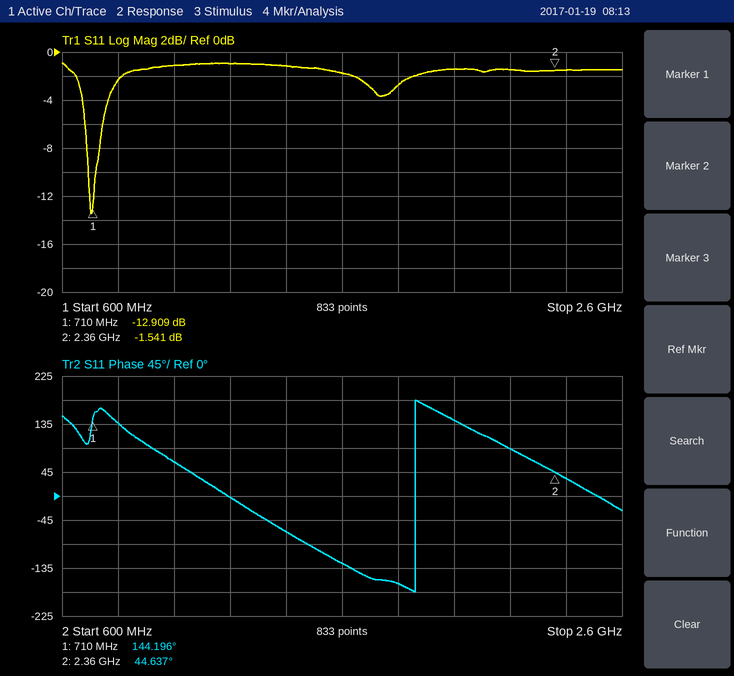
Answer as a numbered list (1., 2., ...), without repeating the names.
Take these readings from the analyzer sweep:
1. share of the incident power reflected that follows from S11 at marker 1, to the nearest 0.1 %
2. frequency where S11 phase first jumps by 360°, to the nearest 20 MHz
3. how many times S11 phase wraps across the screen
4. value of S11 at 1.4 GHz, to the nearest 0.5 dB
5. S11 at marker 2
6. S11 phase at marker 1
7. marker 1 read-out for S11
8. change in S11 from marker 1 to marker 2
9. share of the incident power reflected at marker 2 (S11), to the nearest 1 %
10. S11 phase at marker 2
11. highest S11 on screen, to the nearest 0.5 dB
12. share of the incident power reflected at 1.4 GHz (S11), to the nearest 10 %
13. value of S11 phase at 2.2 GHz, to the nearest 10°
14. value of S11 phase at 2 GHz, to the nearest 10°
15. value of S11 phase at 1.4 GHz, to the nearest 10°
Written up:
1. 5.1 %
2. 1.86 GHz
3. 1
4. -1.0 dB
5. -1.541 dB
6. 144.196°
7. -12.909 dB
8. 11.368 dB
9. 70 %
10. 44.637°
11. -1.0 dB
12. 80 %
13. 90°
14. 140°
15. -70°
